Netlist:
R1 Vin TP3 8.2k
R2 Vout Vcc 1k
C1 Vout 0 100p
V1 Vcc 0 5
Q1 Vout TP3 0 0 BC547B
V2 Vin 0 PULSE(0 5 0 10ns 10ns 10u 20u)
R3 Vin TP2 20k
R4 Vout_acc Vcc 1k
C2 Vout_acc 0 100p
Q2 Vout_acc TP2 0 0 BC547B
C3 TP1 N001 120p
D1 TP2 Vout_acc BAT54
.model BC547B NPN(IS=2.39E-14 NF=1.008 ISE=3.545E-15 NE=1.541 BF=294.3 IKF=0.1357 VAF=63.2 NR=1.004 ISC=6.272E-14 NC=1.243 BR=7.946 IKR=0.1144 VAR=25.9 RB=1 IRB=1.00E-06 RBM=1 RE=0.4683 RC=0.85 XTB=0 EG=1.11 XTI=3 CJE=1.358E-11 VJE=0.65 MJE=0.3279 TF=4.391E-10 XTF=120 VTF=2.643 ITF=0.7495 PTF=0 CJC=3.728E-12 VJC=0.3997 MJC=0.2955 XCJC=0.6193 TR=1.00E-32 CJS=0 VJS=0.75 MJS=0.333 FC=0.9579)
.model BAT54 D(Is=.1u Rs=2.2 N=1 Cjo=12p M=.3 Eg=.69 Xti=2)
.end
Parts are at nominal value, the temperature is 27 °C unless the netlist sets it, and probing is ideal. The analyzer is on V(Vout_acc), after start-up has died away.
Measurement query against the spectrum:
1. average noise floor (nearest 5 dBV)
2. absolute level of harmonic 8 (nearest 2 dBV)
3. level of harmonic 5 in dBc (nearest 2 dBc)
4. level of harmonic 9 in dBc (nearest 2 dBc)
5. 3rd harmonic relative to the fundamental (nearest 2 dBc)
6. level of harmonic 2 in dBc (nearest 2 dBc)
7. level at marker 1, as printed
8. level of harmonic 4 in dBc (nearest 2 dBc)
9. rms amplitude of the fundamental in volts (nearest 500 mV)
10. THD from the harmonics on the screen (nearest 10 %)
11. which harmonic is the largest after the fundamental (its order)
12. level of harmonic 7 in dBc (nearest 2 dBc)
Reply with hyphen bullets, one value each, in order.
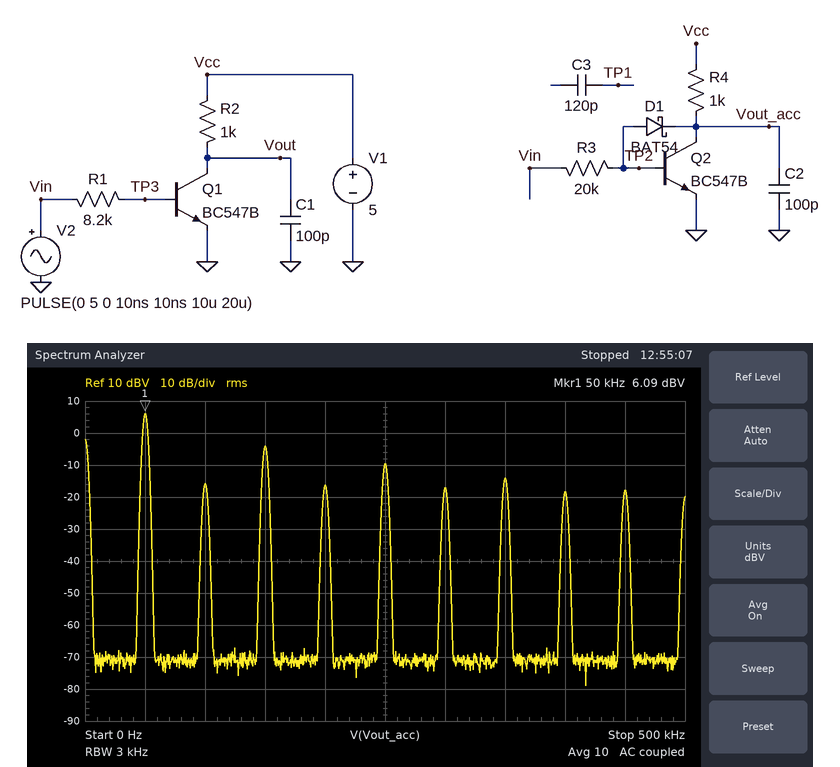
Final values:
- -70 dBV
- -18 dBV
- -16 dBc
- -24 dBc
- -10 dBc
- -22 dBc
- 6.09 dBV
- -22 dBc
- 2.0 V
- 40 %
- 3
- -20 dBc
